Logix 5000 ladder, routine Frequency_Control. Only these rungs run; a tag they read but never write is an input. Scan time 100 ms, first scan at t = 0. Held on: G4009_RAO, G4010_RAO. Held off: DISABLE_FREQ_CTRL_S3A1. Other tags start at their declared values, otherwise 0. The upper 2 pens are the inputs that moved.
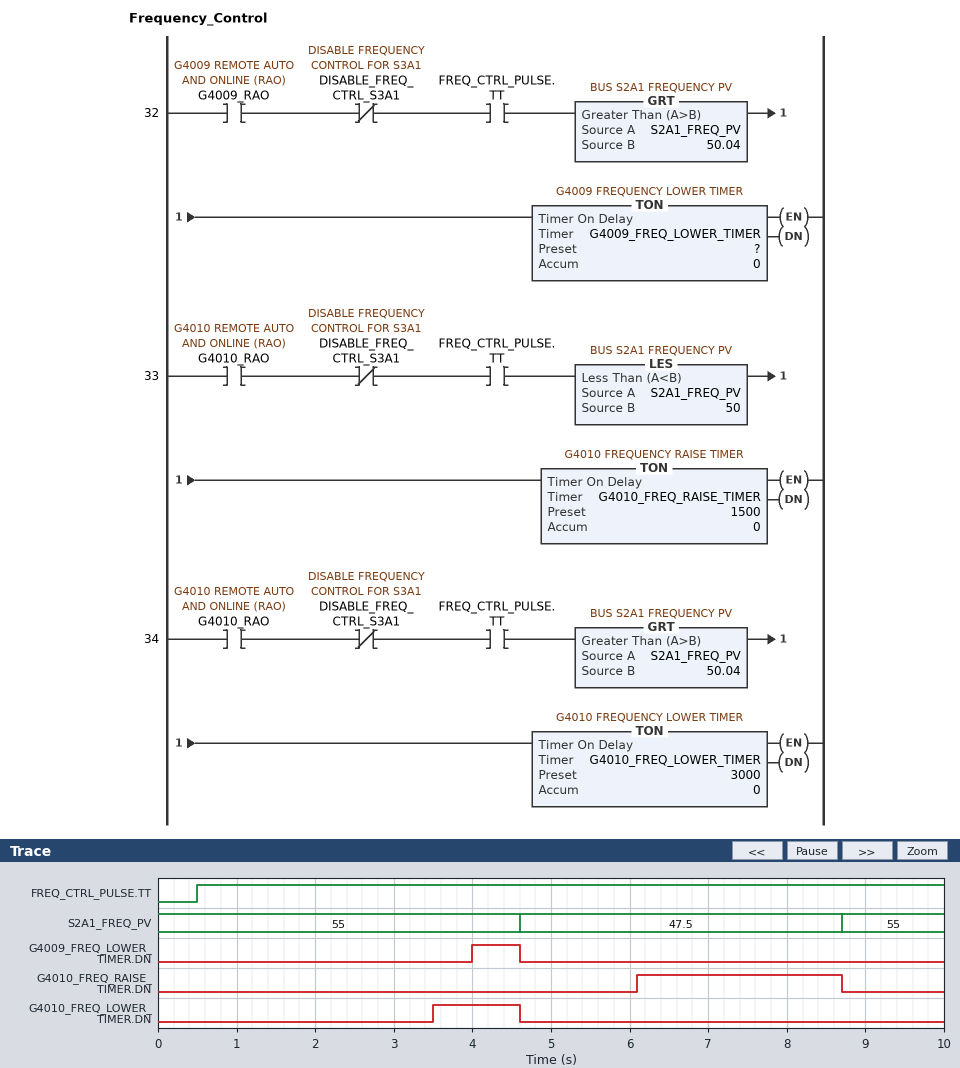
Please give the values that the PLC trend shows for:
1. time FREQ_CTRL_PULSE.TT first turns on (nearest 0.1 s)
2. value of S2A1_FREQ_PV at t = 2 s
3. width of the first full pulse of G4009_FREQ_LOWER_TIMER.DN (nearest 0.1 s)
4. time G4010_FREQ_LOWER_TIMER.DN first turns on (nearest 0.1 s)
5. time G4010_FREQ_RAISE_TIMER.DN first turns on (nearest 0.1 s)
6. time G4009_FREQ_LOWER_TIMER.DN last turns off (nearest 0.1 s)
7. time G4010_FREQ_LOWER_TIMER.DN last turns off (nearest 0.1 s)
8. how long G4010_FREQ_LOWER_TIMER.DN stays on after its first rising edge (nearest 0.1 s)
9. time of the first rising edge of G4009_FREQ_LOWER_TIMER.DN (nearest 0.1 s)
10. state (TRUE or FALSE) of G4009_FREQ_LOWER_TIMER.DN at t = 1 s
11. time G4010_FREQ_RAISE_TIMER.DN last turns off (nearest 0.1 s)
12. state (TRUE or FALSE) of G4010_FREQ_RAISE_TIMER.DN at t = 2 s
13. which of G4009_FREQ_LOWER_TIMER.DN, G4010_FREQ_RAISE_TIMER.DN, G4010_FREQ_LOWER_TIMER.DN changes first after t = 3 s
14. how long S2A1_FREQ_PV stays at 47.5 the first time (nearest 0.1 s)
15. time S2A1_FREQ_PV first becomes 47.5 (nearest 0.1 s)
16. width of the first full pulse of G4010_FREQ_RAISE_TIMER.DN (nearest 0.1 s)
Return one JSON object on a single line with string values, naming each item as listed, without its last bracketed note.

{"time FREQ_CTRL_PULSE.TT first turns on": "0.5 s", "value of S2A1_FREQ_PV at t = 2 s": "55", "width of the first full pulse of G4009_FREQ_LOWER_TIMER.DN": "0.6 s", "time G4010_FREQ_LOWER_TIMER.DN first turns on": "3.5 s", "time G4010_FREQ_RAISE_TIMER.DN first turns on": "6.1 s", "time G4009_FREQ_LOWER_TIMER.DN last turns off": "4.6 s", "time G4010_FREQ_LOWER_TIMER.DN last turns off": "4.6 s", "how long G4010_FREQ_LOWER_TIMER.DN stays on after its first rising edge": "1.1 s", "time of the first rising edge of G4009_FREQ_LOWER_TIMER.DN": "4.0 s", "state (TRUE or FALSE) of G4009_FREQ_LOWER_TIMER.DN at t = 1 s": "FALSE", "time G4010_FREQ_RAISE_TIMER.DN last turns off": "8.7 s", "state (TRUE or FALSE) of G4010_FREQ_RAISE_TIMER.DN at t = 2 s": "FALSE", "which of G4009_FREQ_LOWER_TIMER.DN, G4010_FREQ_RAISE_TIMER.DN, G4010_FREQ_LOWER_TIMER.DN changes first after t = 3 s": "G4010_FREQ_LOWER_TIMER.DN", "how long S2A1_FREQ_PV stays at 47.5 the first time": "4.1 s", "time S2A1_FREQ_PV first becomes 47.5": "4.6 s", "width of the first full pulse of G4010_FREQ_RAISE_TIMER.DN": "2.6 s"}
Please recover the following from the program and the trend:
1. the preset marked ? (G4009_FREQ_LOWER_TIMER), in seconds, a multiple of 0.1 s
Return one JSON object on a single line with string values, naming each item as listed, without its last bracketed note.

{"the preset marked ? (G4009_FREQ_LOWER_TIMER), in seconds, a multiple of 0.1 s": "3.5 s"}
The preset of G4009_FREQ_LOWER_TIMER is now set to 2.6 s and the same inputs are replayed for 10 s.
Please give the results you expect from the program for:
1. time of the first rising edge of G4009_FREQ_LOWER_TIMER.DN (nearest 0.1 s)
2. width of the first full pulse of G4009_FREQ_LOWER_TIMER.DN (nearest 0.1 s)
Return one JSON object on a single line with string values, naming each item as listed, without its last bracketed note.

{"time of the first rising edge of G4009_FREQ_LOWER_TIMER.DN": "3.1 s", "width of the first full pulse of G4009_FREQ_LOWER_TIMER.DN": "1.5 s"}
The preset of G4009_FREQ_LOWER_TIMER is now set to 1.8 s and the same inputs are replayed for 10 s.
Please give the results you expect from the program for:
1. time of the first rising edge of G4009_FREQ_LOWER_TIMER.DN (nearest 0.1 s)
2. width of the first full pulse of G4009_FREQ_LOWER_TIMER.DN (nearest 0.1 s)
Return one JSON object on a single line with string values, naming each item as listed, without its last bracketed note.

{"time of the first rising edge of G4009_FREQ_LOWER_TIMER.DN": "2.3 s", "width of the first full pulse of G4009_FREQ_LOWER_TIMER.DN": "2.3 s"}
